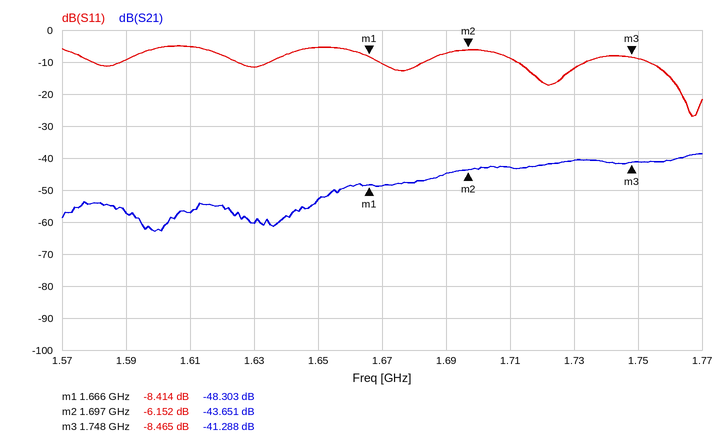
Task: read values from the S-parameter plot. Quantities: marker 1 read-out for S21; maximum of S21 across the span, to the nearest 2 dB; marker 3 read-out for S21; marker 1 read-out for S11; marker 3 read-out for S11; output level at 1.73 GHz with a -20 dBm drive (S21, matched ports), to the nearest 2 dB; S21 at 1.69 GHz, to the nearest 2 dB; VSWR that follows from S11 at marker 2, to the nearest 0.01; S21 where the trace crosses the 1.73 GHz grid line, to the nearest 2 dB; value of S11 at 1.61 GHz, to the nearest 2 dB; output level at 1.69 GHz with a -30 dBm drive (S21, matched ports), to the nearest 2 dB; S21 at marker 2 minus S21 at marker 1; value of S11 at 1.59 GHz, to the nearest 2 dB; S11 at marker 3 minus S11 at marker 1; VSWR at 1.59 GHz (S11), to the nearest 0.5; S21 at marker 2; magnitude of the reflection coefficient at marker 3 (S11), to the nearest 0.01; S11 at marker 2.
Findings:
-48.303 dB
-38 dB
-41.288 dB
-8.414 dB
-8.465 dB
-60 dBm
-44 dB
2.94
-40 dB
-6 dB
-74 dBm
4.652 dB
-10 dB
-0.051 dB
2.0
-43.651 dB
0.38
-6.152 dB
